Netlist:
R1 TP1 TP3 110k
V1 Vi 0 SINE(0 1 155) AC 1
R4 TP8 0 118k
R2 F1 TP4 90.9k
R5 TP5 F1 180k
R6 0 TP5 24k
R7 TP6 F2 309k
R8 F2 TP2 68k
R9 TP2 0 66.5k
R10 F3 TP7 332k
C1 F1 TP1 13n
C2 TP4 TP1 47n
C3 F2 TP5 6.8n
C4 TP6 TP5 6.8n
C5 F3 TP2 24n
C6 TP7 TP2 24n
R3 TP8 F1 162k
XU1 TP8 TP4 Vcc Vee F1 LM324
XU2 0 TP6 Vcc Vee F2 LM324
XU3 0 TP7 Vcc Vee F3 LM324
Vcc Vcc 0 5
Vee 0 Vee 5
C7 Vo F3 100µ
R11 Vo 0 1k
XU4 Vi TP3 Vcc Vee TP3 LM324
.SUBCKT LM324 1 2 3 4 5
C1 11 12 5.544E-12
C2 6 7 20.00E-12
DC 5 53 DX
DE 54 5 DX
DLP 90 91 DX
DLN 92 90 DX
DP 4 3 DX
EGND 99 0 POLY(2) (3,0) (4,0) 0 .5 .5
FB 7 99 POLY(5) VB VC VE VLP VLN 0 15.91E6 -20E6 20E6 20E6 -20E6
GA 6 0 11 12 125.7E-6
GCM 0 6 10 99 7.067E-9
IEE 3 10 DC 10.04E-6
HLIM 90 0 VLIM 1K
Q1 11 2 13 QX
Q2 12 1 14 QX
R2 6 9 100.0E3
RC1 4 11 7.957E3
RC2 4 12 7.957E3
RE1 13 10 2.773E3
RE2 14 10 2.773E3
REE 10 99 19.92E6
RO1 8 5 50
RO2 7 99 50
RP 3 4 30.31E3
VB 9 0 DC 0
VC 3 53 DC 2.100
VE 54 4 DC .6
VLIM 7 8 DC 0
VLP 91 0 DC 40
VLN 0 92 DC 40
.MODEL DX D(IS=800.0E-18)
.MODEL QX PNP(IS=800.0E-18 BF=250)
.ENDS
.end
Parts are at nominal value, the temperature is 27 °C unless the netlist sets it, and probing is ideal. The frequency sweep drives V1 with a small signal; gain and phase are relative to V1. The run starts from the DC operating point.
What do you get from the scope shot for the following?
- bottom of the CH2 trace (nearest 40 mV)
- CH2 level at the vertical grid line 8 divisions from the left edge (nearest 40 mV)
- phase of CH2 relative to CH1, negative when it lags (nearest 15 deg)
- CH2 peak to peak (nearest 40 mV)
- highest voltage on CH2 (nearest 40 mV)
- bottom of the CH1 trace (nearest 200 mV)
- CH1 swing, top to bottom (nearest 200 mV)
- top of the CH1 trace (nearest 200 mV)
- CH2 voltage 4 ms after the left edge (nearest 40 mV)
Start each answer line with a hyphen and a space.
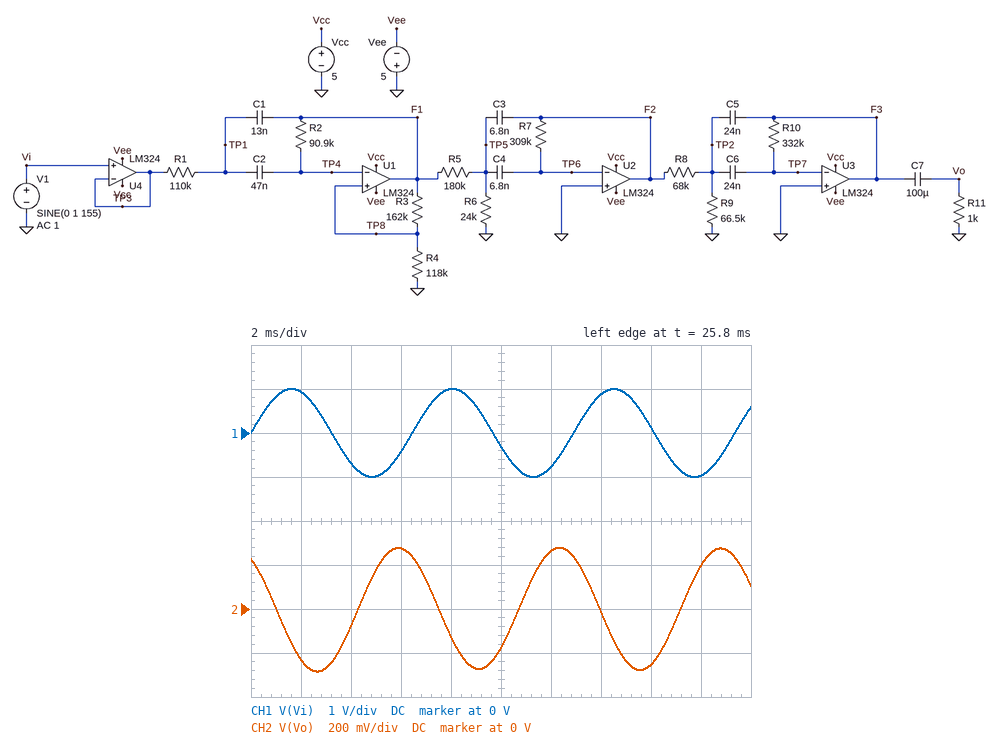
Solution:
- -280 mV
- -240 mV
- 120 deg
- 560 mV
- 280 mV
- -1.0 V
- 2.0 V
- 1.0 V
- -80 mV
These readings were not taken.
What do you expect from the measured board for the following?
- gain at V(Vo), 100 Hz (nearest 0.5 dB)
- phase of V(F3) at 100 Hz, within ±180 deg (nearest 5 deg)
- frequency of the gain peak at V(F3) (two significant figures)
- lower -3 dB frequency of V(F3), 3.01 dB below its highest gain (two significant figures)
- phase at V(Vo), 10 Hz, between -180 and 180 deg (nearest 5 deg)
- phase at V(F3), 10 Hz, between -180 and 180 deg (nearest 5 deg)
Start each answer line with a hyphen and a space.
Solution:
- -7.5 dB
- 170 deg
- 70 Hz
- 54 Hz
- 80 deg
- 70 deg
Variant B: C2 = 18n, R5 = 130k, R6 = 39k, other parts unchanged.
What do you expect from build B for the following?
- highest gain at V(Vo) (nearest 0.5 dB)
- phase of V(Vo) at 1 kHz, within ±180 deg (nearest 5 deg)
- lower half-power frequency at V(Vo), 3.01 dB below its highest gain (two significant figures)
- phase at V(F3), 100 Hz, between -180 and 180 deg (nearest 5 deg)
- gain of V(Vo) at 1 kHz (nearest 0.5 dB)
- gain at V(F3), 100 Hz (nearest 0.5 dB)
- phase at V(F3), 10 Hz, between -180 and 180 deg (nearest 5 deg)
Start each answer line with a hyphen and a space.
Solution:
- -4.0 dB
- -70 deg
- 59 Hz
- -160 deg
- -49.0 dB
- -4.5 dB
- 75 deg
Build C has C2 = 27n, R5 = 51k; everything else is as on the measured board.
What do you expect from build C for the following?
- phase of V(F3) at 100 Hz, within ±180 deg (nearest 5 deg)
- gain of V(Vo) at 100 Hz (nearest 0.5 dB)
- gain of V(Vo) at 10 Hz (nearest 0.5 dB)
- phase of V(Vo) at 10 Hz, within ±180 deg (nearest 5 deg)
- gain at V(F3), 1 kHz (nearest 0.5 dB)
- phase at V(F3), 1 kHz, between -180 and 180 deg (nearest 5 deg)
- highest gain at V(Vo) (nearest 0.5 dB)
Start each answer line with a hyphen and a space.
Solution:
- -170 deg
- 0 dB
- -51.0 dB
- 85 deg
- -40.5 dB
- -70 deg
- 1.0 dB
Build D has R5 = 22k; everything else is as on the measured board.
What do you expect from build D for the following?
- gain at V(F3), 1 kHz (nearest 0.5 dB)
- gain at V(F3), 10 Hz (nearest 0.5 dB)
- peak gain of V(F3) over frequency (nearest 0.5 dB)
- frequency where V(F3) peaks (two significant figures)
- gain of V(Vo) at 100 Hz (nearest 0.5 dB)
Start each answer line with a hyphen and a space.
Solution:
- -32.5 dB
- -42.0 dB
- 7.5 dB
- 69 Hz
- 5.0 dB
